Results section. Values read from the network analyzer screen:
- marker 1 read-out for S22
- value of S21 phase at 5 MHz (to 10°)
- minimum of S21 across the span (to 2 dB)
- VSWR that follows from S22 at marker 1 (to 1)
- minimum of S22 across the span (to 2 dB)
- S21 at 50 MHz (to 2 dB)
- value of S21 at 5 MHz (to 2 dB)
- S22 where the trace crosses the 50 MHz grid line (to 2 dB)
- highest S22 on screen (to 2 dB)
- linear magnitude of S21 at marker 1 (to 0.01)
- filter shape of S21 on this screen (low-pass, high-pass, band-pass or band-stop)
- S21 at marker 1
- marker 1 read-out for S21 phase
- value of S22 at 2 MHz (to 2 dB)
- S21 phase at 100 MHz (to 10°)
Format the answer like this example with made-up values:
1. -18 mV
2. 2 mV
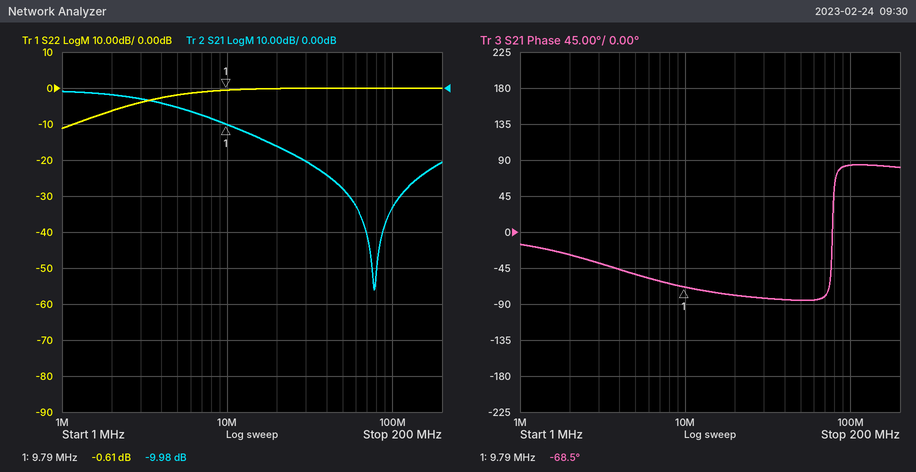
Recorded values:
1. -0.61 dB
2. -50°
3. -56 dB
4. 28
5. -12 dB
6. -28 dB
7. -6 dB
8. 0 dB
9. 0 dB
10. 0.32
11. low-pass
12. -9.98 dB
13. -68.5°
14. -6 dB
15. 80°
